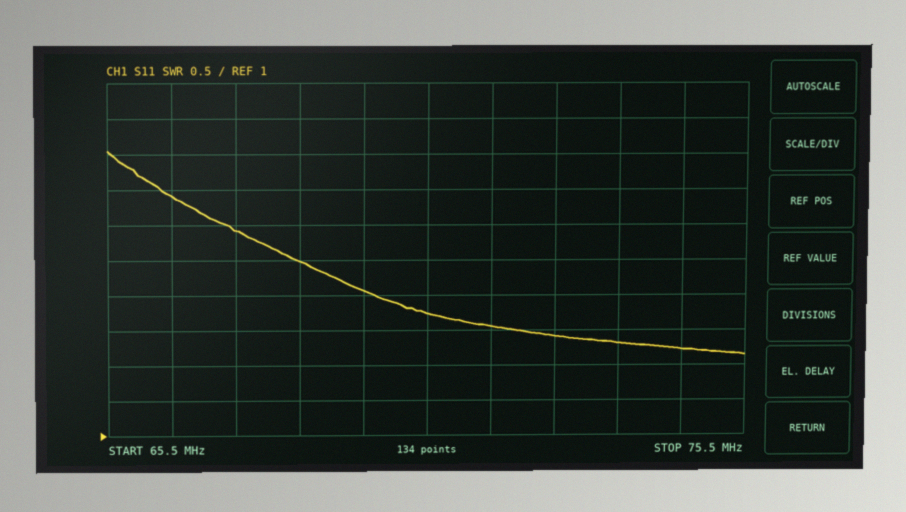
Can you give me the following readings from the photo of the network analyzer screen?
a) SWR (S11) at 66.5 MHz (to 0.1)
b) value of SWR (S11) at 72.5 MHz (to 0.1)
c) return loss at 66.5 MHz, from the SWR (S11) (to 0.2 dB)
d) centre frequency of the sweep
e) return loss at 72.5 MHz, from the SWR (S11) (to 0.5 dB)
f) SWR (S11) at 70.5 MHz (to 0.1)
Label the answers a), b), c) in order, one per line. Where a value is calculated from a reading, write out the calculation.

a) 4.4
b) 2.4
c) −20 log10((4.4 − 1)/(4.4 + 1)) ≈ 4.0 dB
d) 70.5 MHz
e) −20 log10((2.4 − 1)/(2.4 + 1)) ≈ 7.71 dB, so 7.5 dB to the nearest 0.5 dB
f) 2.7
